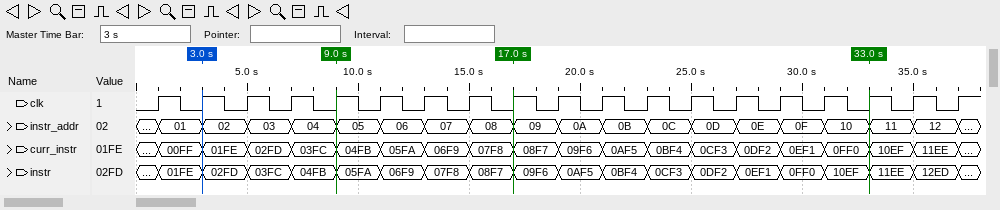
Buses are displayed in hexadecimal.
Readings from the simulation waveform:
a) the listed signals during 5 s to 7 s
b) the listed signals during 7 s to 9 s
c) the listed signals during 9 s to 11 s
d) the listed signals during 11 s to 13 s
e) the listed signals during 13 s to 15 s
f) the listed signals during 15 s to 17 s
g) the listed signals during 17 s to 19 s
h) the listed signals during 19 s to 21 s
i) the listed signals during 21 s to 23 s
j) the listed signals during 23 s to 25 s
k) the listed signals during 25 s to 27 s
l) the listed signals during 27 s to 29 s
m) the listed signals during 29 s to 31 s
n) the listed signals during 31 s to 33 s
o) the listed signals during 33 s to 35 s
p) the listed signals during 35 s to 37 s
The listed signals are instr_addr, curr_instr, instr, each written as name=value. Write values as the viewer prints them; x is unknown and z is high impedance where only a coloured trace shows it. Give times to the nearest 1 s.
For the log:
instr_addr=03, curr_instr=02FD, instr=03FC
instr_addr=04, curr_instr=03FC, instr=04FB
instr_addr=05, curr_instr=04FB, instr=05FA
instr_addr=06, curr_instr=05FA, instr=06F9
instr_addr=07, curr_instr=06F9, instr=07F8
instr_addr=08, curr_instr=07F8, instr=08F7
instr_addr=09, curr_instr=08F7, instr=09F6
instr_addr=0A, curr_instr=09F6, instr=0AF5
instr_addr=0B, curr_instr=0AF5, instr=0BF4
instr_addr=0C, curr_instr=0BF4, instr=0CF3
instr_addr=0D, curr_instr=0CF3, instr=0DF2
instr_addr=0E, curr_instr=0DF2, instr=0EF1
instr_addr=0F, curr_instr=0EF1, instr=0FF0
instr_addr=10, curr_instr=0FF0, instr=10EF
instr_addr=11, curr_instr=10EF, instr=11EE
instr_addr=12, curr_instr=11EE, instr=12ED
